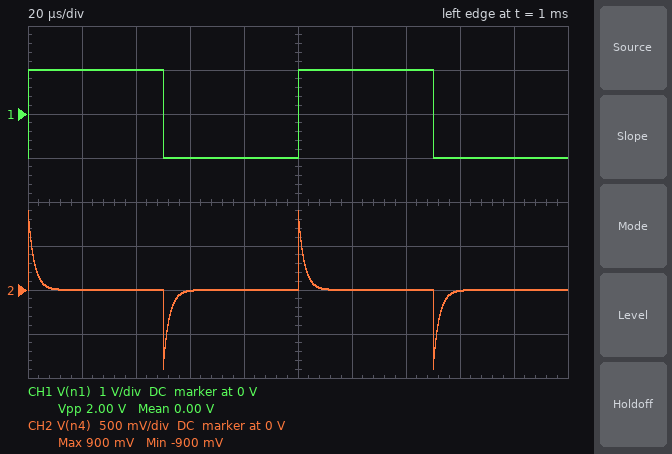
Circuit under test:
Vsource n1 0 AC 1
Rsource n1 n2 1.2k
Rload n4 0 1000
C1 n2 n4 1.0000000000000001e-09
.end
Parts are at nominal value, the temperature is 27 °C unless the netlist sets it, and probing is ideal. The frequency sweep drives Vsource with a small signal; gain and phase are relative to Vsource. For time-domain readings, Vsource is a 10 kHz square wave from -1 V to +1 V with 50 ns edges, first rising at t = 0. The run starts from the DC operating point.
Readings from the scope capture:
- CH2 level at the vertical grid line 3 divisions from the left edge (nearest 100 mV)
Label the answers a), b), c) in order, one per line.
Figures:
a) 0 V
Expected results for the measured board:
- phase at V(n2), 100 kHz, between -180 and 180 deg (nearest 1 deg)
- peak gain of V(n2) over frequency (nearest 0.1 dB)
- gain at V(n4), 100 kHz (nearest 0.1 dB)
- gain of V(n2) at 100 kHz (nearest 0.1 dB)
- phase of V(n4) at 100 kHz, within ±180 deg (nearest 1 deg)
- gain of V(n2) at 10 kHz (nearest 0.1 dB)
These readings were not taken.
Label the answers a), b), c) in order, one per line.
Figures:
a) -22 deg
b) 0 dB
c) -8.7 dB
d) -3.2 dB
e) 36 deg
f) -0.1 dB
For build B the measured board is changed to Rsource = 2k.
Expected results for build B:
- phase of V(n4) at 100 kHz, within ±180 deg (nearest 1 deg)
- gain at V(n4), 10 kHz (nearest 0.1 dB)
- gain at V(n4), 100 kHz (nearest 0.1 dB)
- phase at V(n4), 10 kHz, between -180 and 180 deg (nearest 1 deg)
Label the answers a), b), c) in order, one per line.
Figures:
a) 28 deg
b) -24.2 dB
c) -10.6 dB
d) 79 deg
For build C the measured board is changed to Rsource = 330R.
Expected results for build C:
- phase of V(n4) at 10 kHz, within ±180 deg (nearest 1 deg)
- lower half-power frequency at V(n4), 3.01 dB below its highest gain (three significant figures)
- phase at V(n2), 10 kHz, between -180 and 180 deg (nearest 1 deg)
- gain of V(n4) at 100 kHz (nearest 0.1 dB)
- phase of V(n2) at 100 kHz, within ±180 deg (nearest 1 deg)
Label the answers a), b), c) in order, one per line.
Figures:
a) 85 deg
b) 120 kHz
c) -1 deg
d) -6.3 dB
e) -8 deg
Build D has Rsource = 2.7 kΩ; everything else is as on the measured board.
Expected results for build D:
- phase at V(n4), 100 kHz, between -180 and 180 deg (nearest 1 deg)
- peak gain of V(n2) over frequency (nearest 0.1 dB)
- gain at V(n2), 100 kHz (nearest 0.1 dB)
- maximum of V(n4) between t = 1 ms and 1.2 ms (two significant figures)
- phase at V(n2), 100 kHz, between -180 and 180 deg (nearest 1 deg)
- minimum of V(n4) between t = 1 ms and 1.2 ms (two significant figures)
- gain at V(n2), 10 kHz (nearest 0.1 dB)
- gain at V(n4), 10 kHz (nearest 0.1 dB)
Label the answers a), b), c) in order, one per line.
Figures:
a) 23 deg
b) 0 dB
c) -6.6 dB
d) 540 mV
e) -35 deg
f) -540 mV
g) -0.2 dB
h) -24.3 dB
